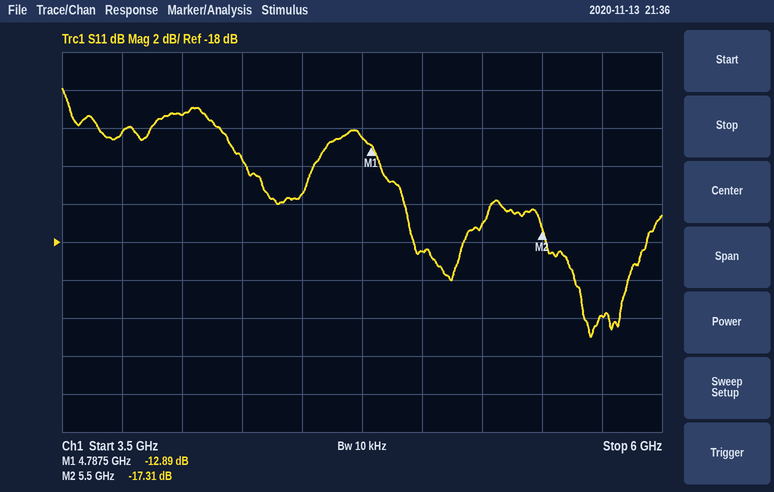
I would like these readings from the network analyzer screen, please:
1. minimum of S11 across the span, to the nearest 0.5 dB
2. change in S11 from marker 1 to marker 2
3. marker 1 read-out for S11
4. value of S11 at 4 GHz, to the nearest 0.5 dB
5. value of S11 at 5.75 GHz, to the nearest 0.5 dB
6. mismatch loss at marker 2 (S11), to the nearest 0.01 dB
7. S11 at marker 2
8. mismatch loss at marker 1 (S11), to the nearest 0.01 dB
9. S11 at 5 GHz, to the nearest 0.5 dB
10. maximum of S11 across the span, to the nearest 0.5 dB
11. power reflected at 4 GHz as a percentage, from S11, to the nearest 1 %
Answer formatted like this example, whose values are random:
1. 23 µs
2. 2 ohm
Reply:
1. -23.0 dB
2. -4.42 dB
3. -12.89 dB
4. -11.5 dB
5. -22.0 dB
6. 0.08 dB
7. -17.31 dB
8. 0.23 dB
9. -18.5 dB
10. -10.0 dB
11. 7 %
